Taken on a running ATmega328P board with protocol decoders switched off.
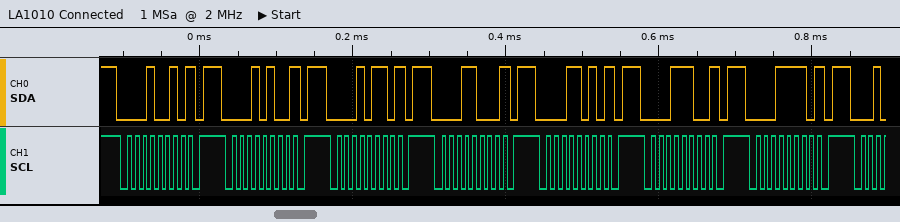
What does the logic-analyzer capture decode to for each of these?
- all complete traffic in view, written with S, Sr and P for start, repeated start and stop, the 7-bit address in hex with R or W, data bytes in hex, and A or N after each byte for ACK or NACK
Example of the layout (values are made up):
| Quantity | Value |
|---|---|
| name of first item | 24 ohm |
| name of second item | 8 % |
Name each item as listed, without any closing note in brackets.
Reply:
| Quantity | Value |
|---|---|
| all complete traffic in view, written with S, Sr and P for start, repeated start and stop, the 7-bit address in hex with R or W, data bytes in hex, and A or N after each byte for ACK or NACK | S 09W N P S 0AW N P S 0BW N P S 0CW N P S 0DW N P S 0EW N P S 0FW N P |
